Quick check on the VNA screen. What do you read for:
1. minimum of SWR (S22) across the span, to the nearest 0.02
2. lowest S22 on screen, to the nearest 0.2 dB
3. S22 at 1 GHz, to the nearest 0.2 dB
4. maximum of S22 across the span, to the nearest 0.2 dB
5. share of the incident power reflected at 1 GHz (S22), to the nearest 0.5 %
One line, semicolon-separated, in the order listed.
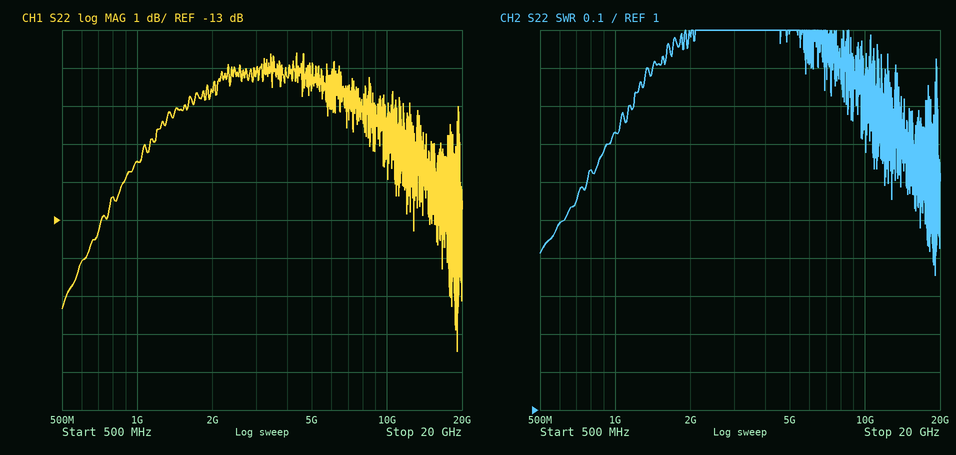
1.36; -16.4 dB; -11.4 dB; -8.6 dB; 7.0 %
